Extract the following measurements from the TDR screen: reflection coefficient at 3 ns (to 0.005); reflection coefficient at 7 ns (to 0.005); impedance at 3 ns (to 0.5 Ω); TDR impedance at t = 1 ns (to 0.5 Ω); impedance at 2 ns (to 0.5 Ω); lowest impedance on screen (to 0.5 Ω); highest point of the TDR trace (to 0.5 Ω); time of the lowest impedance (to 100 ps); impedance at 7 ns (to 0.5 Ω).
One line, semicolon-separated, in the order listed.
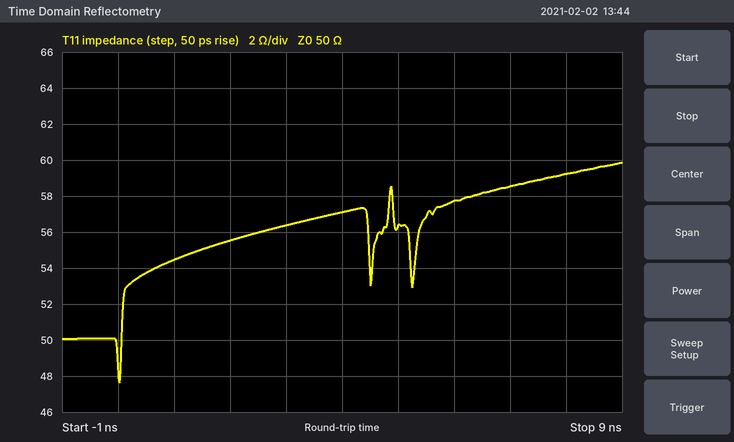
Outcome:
+0.060; +0.080; 56.5 Ω; 54.5 Ω; 55.5 Ω; 47.5 Ω; 60.0 Ω; 0.0 ns; 58.5 Ω
